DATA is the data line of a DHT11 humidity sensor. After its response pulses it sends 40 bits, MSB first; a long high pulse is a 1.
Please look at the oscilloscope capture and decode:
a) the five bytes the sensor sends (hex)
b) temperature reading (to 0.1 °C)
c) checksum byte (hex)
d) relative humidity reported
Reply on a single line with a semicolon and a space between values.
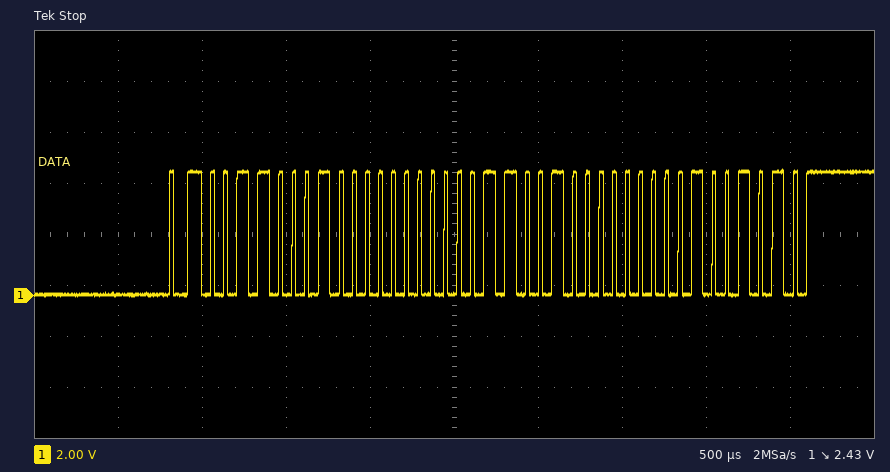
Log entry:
31 00 19 00 4A; 25.0 °C; 0x4A; 49 %
